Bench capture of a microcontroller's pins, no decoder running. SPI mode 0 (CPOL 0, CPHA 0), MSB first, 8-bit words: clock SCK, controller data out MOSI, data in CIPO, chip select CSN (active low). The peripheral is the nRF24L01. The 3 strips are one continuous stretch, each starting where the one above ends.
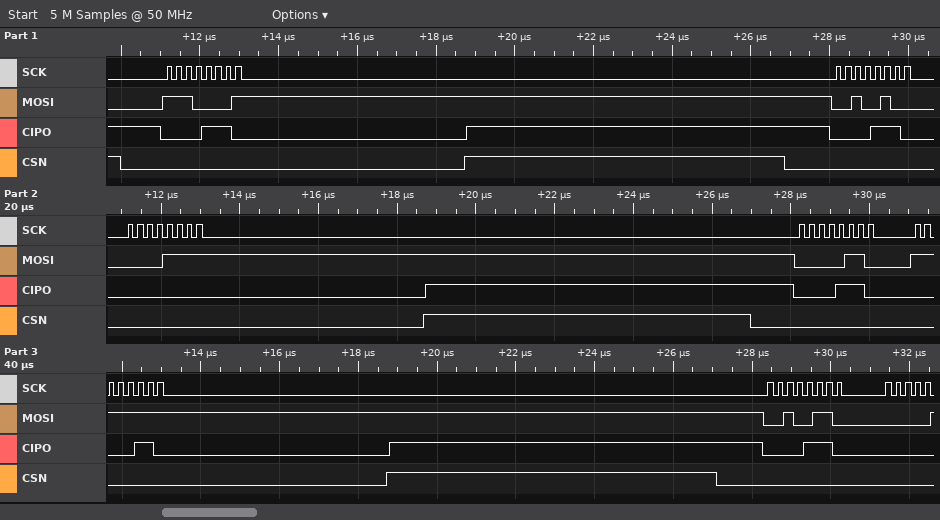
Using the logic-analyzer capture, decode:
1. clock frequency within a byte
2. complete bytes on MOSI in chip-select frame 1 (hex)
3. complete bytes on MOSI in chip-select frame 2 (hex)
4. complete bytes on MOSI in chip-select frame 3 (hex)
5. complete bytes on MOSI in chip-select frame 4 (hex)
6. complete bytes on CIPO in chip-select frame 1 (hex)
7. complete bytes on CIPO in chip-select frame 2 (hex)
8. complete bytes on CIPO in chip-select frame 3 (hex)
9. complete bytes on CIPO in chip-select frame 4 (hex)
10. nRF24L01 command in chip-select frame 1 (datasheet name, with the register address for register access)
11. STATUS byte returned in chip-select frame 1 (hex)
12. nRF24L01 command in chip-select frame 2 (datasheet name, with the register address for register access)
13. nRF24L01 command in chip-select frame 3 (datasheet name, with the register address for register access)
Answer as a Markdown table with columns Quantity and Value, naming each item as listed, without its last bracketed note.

| Quantity | Value |
|---|---|
| clock frequency within a byte | 4 MHz |
| complete bytes on MOSI in chip-select frame 1 | 0xE1 |
| complete bytes on MOSI in chip-select frame 2 | 0x24 0x0F |
| complete bytes on MOSI in chip-select frame 3 | 0x06 0xFF |
| complete bytes on MOSI in chip-select frame 4 | 0x26 |
| complete bytes on CIPO in chip-select frame 1 | 0x0E |
| complete bytes on CIPO in chip-select frame 2 | 0x0E 0x00 |
| complete bytes on CIPO in chip-select frame 3 | 0x0E 0x06 |
| complete bytes on CIPO in chip-select frame 4 | 0x0E |
| nRF24L01 command in chip-select frame 1 | FLUSH_TX |
| STATUS byte returned in chip-select frame 1 | 0x0E |
| nRF24L01 command in chip-select frame 2 | W_REGISTER 0x04 |
| nRF24L01 command in chip-select frame 3 | R_REGISTER 0x06 |
